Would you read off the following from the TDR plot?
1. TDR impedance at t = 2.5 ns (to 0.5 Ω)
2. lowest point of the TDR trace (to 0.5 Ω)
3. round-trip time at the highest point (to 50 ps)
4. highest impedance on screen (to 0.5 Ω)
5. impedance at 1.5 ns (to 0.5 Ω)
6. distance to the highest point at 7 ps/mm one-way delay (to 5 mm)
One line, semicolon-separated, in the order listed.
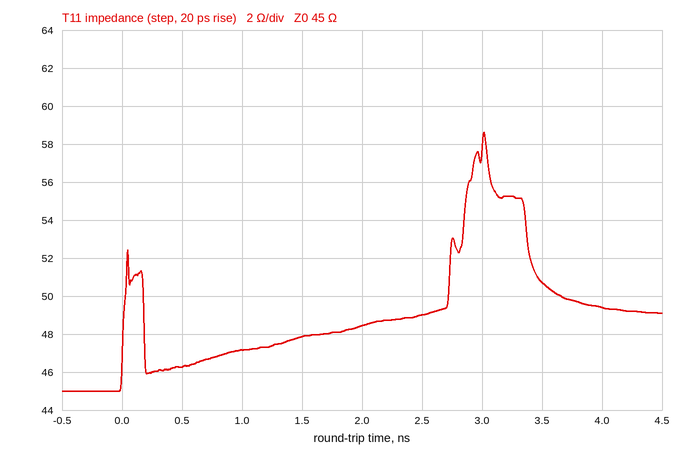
49.0 Ω; 45.0 Ω; 3.00 ns; 58.5 Ω; 48.0 Ω; 215 mm
